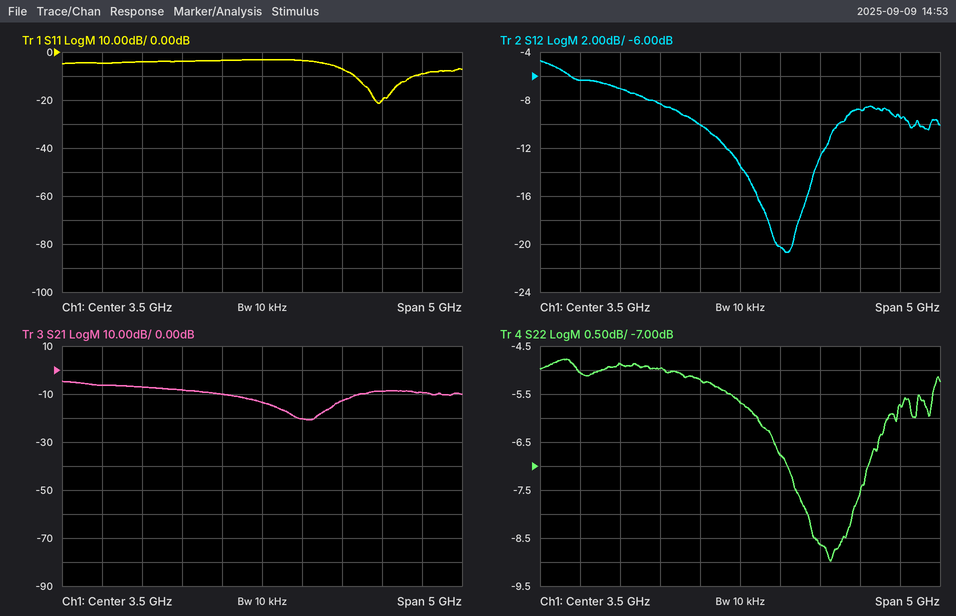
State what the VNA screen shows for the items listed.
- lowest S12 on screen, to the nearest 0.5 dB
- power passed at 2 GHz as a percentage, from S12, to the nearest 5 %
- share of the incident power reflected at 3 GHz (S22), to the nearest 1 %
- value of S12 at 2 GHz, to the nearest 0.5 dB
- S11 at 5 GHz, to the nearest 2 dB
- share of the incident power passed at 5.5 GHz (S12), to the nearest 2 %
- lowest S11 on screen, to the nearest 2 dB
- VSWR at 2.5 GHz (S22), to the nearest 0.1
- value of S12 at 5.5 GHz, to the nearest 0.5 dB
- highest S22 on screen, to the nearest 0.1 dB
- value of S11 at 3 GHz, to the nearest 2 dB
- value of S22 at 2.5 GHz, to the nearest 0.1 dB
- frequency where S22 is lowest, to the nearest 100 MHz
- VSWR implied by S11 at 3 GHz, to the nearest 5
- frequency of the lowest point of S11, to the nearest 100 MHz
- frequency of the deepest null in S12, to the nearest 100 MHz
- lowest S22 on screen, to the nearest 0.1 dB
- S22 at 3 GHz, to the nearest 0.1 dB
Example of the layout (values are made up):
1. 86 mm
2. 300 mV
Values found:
1. -20.5 dB
2. 20 %
3. 30 %
4. -7.0 dB
5. -20 dB
6. 12 %
7. -22 dB
8. 3.6
9. -9.5 dB
10. -4.8 dB
11. -4 dB
12. -5.0 dB
13. 4.6 GHz
14. 5
15. 5.0 GHz
16. 4.1 GHz
17. -9.0 dB
18. -5.2 dB
